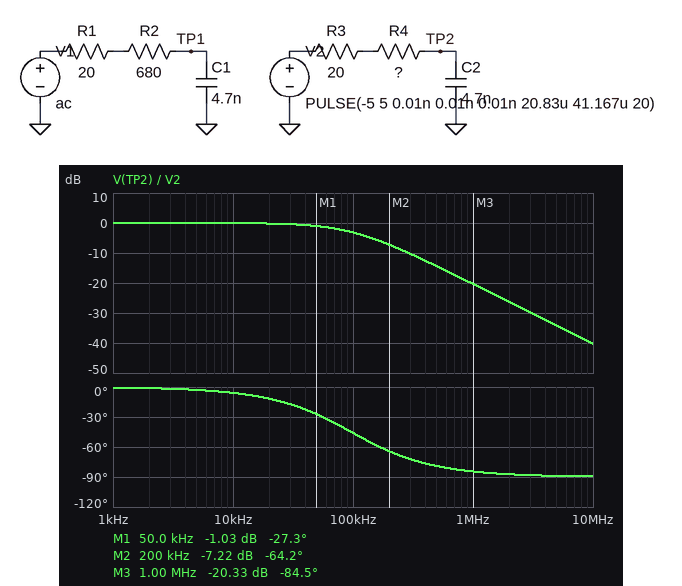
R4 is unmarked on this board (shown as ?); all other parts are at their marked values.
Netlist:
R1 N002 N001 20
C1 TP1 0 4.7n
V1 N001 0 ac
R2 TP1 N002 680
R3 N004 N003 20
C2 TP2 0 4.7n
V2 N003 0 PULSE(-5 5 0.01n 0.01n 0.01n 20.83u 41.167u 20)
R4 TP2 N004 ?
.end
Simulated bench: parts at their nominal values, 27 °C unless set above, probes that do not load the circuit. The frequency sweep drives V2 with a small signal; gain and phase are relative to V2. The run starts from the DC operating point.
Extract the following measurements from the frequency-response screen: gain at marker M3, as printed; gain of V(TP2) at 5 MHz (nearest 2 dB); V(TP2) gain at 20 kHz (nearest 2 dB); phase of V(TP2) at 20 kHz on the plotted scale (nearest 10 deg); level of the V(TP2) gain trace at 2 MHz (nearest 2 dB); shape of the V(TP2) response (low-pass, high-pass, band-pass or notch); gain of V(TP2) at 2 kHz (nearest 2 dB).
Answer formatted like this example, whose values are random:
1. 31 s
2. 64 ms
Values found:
1. -20.33 dB
2. -34 dB
3. 0 dB
4. -10 deg
5. -26 dB
6. low-pass
7. 0 dB
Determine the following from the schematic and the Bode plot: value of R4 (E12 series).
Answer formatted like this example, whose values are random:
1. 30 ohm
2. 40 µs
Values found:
1. 330 Ω
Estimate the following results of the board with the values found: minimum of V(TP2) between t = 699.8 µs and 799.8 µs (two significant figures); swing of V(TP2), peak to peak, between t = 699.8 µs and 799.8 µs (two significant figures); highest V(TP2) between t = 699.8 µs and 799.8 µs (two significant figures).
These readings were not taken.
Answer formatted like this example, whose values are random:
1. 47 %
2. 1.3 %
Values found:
1. -5.0 V
2. 10 V
3. 5.0 V
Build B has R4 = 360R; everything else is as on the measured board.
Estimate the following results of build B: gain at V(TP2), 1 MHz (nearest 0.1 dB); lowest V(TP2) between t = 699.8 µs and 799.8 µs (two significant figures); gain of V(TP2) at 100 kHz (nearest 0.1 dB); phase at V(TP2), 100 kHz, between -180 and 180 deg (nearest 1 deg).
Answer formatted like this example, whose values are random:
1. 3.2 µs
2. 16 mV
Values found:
1. -21.0 dB
2. -5.0 V
3. -3.5 dB
4. -48 deg
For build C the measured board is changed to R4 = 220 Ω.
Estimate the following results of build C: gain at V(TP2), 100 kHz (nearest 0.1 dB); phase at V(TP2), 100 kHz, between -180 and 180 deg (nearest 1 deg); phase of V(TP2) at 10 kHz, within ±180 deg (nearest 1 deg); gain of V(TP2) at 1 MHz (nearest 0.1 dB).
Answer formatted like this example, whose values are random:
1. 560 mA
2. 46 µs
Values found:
1. -1.8 dB
2. -35 deg
3. -4 deg
4. -17.1 dB
